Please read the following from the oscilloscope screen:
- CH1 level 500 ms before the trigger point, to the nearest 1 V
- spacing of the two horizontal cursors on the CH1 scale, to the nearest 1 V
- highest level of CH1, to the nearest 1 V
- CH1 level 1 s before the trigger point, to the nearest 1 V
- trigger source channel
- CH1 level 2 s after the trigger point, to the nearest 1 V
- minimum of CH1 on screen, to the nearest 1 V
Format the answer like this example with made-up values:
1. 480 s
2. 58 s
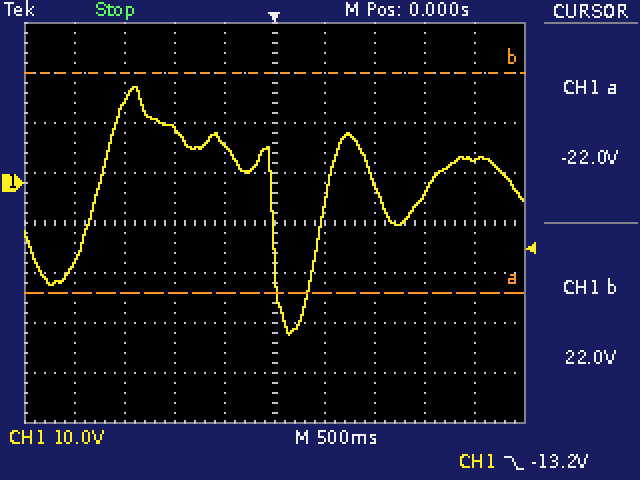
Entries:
1. 8 V
2. 44 V
3. 19 V
4. 11 V
5. CH1
6. 5 V
7. -30 V
